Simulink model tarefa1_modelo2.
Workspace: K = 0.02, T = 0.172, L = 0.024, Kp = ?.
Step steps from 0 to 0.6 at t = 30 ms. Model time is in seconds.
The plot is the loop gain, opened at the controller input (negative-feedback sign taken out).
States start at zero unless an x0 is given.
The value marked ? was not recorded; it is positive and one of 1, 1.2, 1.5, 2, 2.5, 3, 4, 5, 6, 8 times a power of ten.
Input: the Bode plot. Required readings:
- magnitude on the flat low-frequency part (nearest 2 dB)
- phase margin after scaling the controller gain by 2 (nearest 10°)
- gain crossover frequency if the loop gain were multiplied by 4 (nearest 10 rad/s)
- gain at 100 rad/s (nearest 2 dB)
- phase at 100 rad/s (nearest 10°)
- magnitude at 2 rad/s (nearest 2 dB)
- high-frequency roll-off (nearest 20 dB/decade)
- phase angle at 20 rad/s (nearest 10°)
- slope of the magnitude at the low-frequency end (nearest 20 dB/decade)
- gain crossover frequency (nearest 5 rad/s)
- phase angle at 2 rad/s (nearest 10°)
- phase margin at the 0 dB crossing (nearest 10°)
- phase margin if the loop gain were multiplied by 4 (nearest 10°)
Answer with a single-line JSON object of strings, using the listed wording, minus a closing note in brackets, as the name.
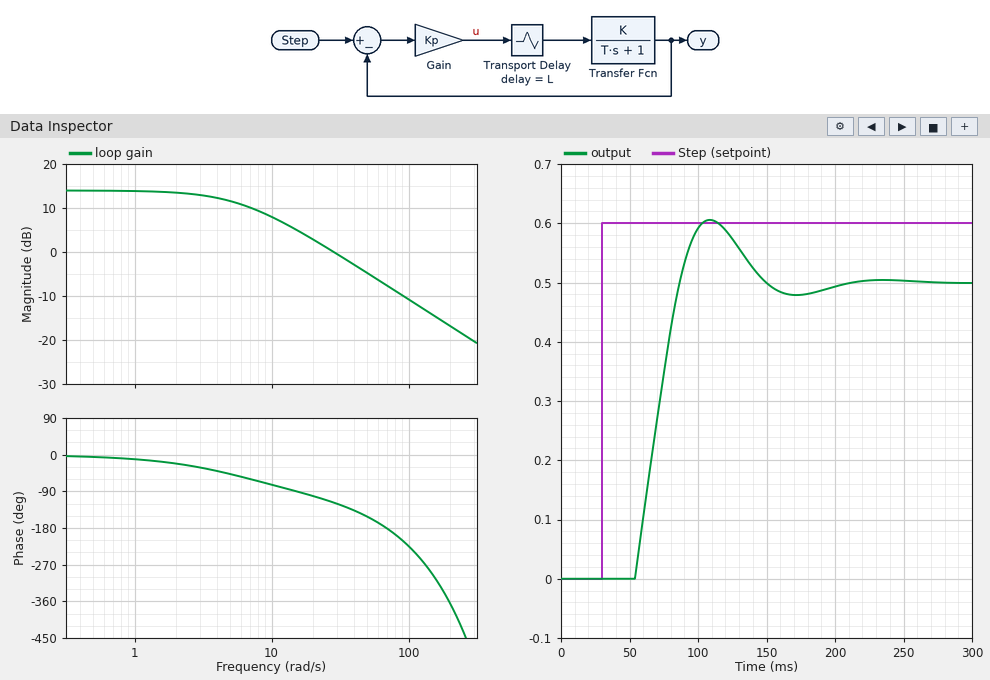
{"magnitude on the flat low-frequency part": "14 dB", "phase margin after scaling the controller gain by 2": "20°", "gain crossover frequency if the loop gain were multiplied by 4": "120 rad/s", "gain at 100 rad/s": "-10 dB", "phase at 100 rad/s": "-220°", "magnitude at 2 rad/s": "14 dB", "high-frequency roll-off": "-20 dB/decade", "phase angle at 20 rad/s": "-100°", "slope of the magnitude at the low-frequency end": "0 dB/decade", "gain crossover frequency": "30 rad/s", "phase angle at 2 rad/s": "-20°", "phase margin at the 0 dB crossing": "60°", "phase margin if the loop gain were multiplied by 4": "-70°"}
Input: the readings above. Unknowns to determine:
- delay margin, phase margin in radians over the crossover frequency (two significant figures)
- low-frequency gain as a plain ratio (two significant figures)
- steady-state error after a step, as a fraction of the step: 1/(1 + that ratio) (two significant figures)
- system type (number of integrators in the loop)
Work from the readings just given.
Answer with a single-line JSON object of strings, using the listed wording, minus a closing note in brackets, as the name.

{"delay margin, phase margin in radians over the crossover frequency": "0.035 s", "low-frequency gain as a plain ratio": "5.0", "steady-state error after a step, as a fraction of the step: 1/(1 + that ratio)": "0.17", "system type": "0"}
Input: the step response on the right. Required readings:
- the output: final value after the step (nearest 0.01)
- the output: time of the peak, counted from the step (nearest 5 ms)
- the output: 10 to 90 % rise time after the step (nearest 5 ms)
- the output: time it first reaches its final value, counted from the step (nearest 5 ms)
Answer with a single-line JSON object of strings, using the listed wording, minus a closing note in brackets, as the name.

{"the output: final value after the step": "0.50", "the output: time of the peak, counted from the step": "80 ms", "the output: 10 to 90 % rise time after the step": "25 ms", "the output: time it first reaches its final value, counted from the step": "55 ms"}
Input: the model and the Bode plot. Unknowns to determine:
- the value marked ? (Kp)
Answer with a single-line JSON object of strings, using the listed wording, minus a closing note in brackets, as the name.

{"the value marked ?": "250"}
